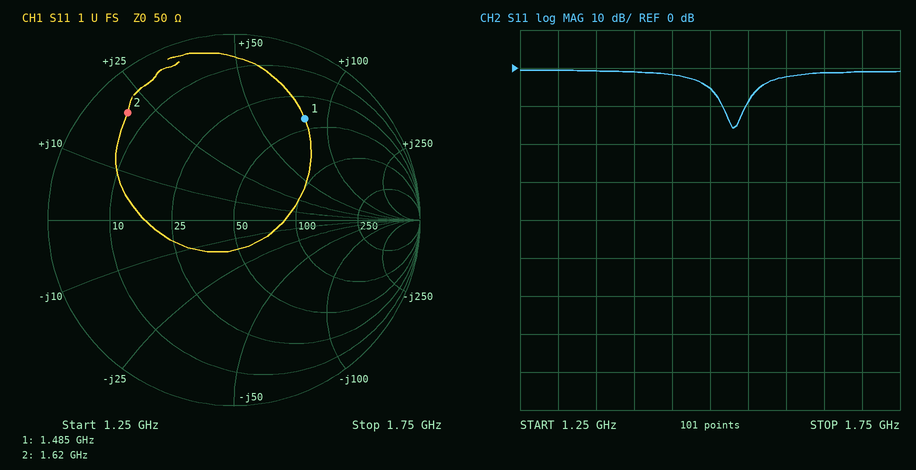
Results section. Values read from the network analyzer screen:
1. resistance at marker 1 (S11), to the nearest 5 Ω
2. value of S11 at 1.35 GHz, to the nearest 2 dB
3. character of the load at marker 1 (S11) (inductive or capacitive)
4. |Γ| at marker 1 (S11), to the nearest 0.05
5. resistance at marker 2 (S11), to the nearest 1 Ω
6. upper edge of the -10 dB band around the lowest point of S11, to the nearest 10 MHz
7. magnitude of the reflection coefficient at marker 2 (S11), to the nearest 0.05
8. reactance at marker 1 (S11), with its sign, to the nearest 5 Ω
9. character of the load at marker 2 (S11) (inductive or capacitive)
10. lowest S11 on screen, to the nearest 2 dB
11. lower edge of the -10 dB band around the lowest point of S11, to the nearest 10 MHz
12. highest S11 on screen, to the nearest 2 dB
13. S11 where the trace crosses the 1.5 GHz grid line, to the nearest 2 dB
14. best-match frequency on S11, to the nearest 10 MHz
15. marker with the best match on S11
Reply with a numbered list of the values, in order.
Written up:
1. 40 Ω
2. 0 dB
3. inductive
4. 0.65
5. 6 Ω
6. 1.55 GHz
7. 0.80
8. +80 Ω
9. inductive
10. -16 dB
11. 1.52 GHz
12. 0 dB
13. -6 dB
14. 1.53 GHz
15. marker 1
